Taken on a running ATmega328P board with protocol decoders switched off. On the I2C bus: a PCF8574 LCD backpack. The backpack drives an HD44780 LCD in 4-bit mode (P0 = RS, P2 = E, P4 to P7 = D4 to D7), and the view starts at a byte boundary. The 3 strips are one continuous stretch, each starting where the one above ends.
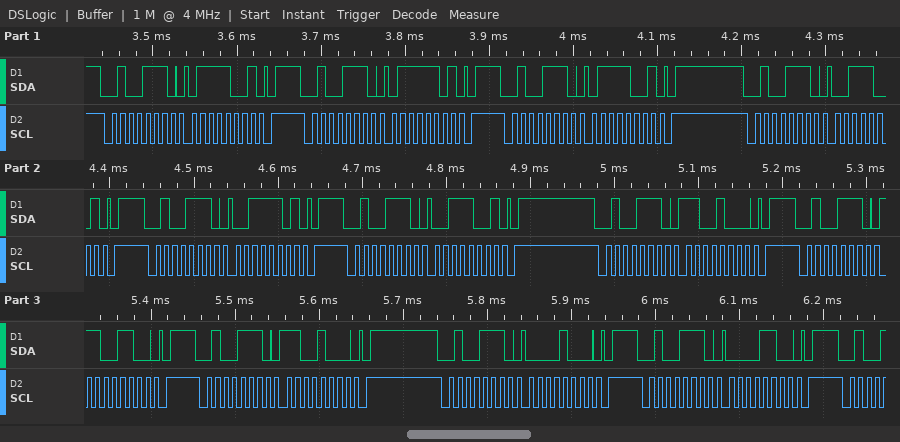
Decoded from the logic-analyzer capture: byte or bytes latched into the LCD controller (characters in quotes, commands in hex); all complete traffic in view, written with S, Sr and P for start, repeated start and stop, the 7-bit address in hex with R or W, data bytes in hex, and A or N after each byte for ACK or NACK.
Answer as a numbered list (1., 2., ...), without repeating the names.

1. 's'
2. S 27W A 79 A P S 27W A 7D A P S 27W A 79 A P S 27W A 39 A P S 27W A 3D A P S 27W A 39 A P S 27W A C8 A P S 27W A CC A P S 27W A C8 A P S 27W A 08 A P S 27W A 0C A P
